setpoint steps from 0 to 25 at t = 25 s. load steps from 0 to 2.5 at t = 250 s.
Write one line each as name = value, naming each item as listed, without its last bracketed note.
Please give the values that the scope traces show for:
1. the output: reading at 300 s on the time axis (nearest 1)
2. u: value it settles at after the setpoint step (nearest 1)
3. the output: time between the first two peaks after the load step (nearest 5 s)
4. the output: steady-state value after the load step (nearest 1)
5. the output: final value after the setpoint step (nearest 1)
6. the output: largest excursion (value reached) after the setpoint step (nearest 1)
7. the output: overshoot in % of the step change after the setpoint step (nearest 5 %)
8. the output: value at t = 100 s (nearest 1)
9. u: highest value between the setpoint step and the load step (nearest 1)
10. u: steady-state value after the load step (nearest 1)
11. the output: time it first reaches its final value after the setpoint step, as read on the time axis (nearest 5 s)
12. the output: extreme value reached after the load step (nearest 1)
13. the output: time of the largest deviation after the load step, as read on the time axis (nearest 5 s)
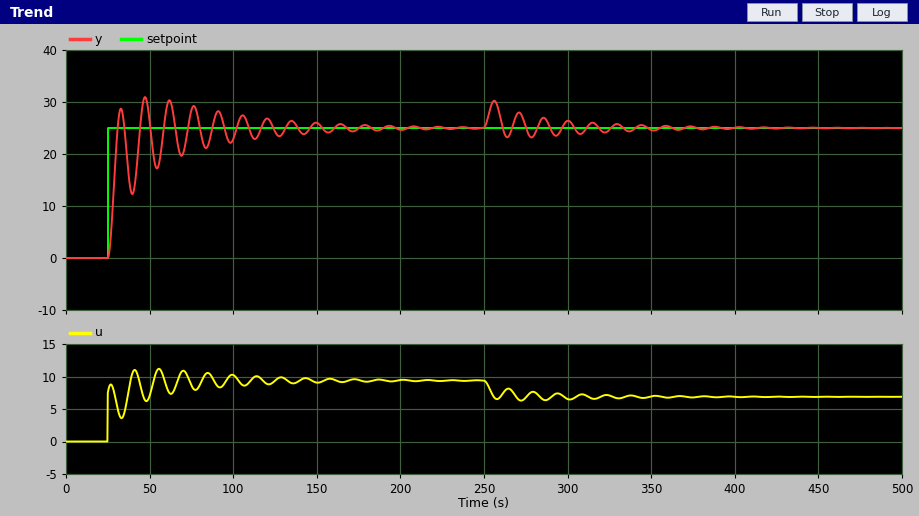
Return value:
the output: reading at 300 s on the time axis = 26
u: value it settles at after the setpoint step = 9
the output: time between the first two peaks after the load step = 15 s
the output: steady-state value after the load step = 25
the output: final value after the setpoint step = 25
the output: largest excursion (value reached) after the setpoint step = 31
the output: overshoot in % of the step change after the setpoint step = 25 %
the output: value at t = 100 s = 23
u: highest value between the setpoint step and the load step = 11
u: steady-state value after the load step = 7
the output: time it first reaches its final value after the setpoint step, as read on the time axis = 30 s
the output: extreme value reached after the load step = 30
the output: time of the largest deviation after the load step, as read on the time axis = 255 s
